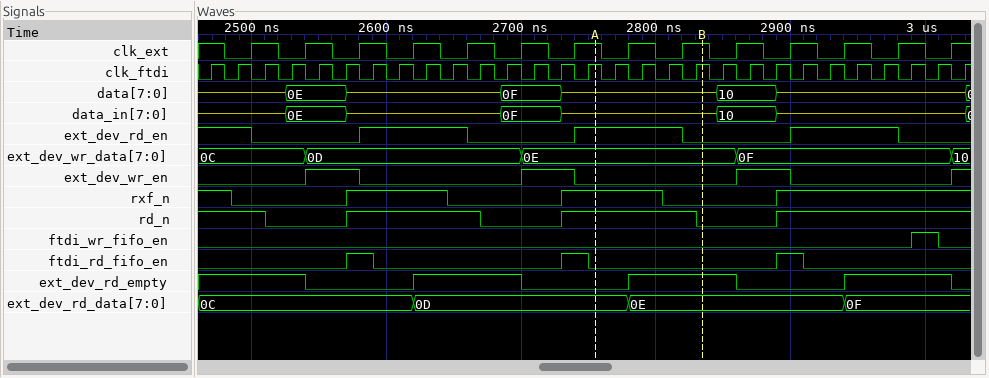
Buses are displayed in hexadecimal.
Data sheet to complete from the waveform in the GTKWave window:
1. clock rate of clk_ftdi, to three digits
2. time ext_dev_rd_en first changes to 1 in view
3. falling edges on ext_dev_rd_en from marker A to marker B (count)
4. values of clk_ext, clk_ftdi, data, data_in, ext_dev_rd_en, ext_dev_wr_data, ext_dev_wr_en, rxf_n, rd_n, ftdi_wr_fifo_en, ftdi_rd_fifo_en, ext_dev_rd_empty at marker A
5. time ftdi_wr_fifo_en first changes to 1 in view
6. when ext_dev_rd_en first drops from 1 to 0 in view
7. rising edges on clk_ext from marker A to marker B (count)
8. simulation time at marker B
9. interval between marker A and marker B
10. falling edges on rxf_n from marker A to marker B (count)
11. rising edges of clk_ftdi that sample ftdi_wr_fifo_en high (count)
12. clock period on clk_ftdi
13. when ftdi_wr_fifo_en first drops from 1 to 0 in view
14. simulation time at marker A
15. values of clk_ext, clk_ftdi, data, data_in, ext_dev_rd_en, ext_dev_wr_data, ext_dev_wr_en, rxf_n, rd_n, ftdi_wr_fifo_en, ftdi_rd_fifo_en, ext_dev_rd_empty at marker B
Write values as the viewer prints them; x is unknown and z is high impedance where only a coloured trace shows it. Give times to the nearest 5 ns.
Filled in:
50.0 MHz
2580 ns
1
clk_ext=1, clk_ftdi=1, data=z, data_in=z, ext_dev_rd_en=1, ext_dev_wr_data=0E, ext_dev_wr_en=0, rxf_n=1, rd_n=1, ftdi_wr_fifo_en=0, ftdi_rd_fifo_en=0, ext_dev_rd_empty=0
2990 ns
2500 ns
2
2835 ns
80 ns
1
1
20 ns
3010 ns
2755 ns
clk_ext=1, clk_ftdi=1, data=z, data_in=z, ext_dev_rd_en=0, ext_dev_wr_data=0E, ext_dev_wr_en=0, rxf_n=0, rd_n=0, ftdi_wr_fifo_en=0, ftdi_rd_fifo_en=0, ext_dev_rd_empty=1
